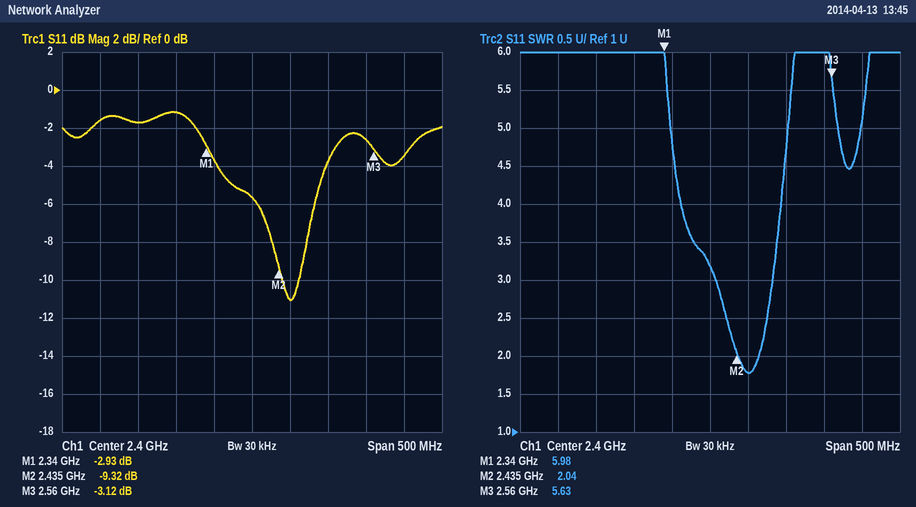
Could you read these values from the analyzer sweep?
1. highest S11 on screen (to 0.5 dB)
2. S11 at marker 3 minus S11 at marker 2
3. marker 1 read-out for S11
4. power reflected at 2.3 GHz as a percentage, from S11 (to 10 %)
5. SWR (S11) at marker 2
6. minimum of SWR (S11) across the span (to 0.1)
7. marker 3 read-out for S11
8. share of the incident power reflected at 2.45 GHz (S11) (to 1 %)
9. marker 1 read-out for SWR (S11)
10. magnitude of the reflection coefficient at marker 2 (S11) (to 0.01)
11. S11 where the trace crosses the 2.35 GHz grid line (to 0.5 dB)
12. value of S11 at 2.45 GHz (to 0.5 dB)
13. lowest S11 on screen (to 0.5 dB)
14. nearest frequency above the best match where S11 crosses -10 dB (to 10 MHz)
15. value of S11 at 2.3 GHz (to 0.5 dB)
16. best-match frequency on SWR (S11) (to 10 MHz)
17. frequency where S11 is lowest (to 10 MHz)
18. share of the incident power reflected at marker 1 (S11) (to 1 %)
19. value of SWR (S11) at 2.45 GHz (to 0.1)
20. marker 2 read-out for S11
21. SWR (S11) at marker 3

-1.0 dB
6.20 dB
-2.93 dB
80 %
2.04
1.8
-3.12 dB
8 %
5.98
0.34
-3.5 dB
-11.0 dB
-11.0 dB
2.46 GHz
-1.0 dB
2.45 GHz
2.45 GHz
51 %
1.8
-9.32 dB
5.63
